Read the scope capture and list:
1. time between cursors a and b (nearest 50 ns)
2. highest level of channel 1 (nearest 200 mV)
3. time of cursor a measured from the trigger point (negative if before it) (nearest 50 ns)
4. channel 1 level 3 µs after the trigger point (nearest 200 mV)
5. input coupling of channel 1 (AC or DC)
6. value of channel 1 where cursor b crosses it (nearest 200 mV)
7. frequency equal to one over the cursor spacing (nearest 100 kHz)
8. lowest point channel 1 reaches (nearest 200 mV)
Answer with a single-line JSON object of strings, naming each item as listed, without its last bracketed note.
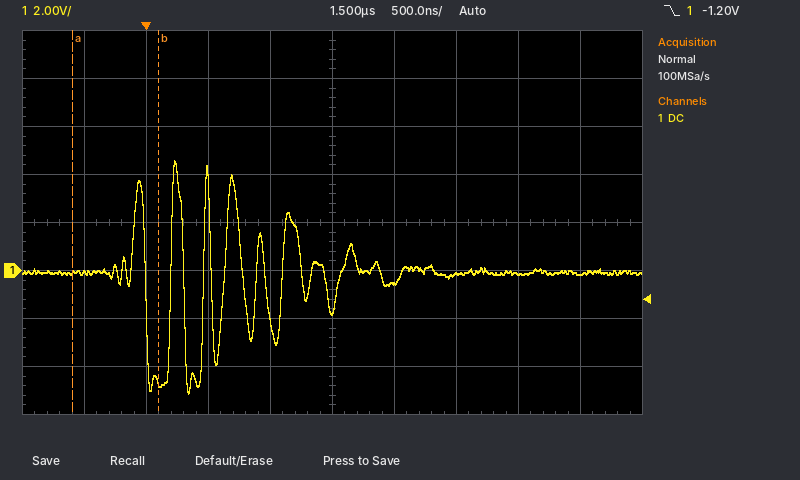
{"time between cursors a and b": "700 ns", "highest level of channel 1": "4.6 V", "time of cursor a measured from the trigger point (negative if before it)": "-600 ns", "channel 1 level 3 µs after the trigger point": "-200 mV", "input coupling of channel 1": "DC", "value of channel 1 where cursor b crosses it": "-4.6 V", "frequency equal to one over the cursor spacing": "1.4 MHz", "lowest point channel 1 reaches": "-5.2 V"}
